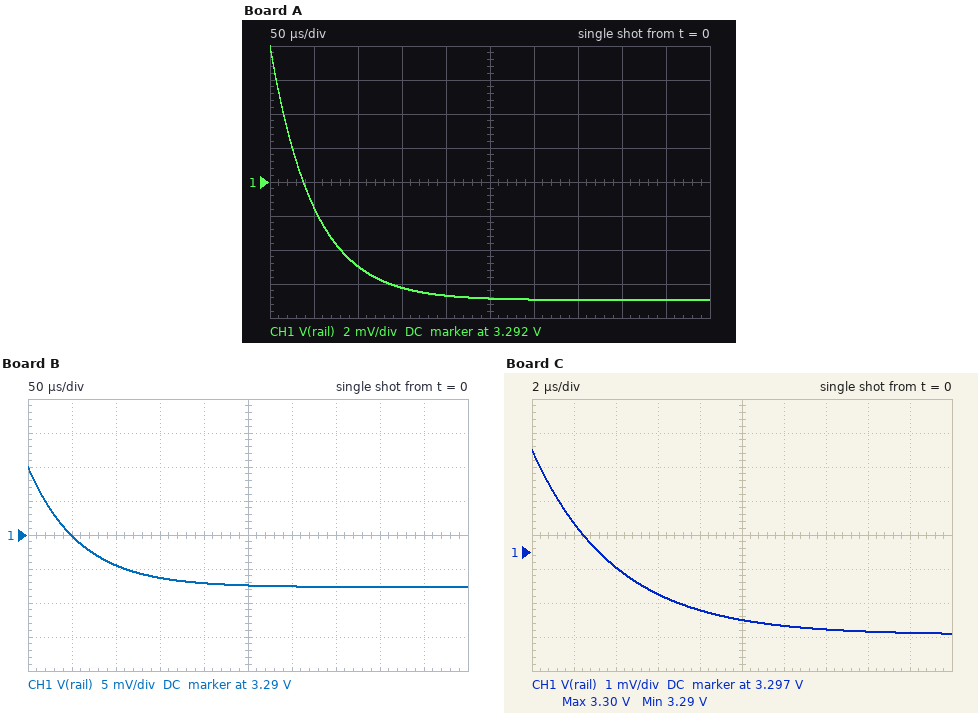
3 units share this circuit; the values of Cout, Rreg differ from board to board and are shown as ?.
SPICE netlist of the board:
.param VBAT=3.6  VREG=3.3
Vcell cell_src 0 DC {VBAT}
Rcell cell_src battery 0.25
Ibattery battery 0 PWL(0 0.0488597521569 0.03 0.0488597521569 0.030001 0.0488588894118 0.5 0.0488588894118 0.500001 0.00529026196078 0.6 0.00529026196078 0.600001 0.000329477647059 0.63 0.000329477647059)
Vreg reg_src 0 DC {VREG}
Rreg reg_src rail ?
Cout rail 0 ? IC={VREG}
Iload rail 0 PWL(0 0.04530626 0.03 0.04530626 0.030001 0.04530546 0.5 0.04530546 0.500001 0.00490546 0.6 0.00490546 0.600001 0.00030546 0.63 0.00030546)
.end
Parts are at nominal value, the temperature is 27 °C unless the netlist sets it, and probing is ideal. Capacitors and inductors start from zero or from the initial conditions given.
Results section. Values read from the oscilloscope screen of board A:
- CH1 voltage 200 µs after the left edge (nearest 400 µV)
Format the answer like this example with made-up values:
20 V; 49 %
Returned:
3.2852 V
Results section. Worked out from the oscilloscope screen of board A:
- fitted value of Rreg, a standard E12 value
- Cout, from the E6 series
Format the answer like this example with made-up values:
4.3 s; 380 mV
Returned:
0.33 Ω; 150 µF
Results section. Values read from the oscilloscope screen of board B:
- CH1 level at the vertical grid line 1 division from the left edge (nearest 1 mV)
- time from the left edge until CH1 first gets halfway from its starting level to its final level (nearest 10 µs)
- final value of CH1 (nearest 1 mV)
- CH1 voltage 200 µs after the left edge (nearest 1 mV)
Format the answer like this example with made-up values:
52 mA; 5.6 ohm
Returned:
3.290 V; 40 µs; 3.282 V; 3.283 V
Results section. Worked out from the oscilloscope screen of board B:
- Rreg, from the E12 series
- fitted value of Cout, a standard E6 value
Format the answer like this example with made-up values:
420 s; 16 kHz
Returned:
0.39 Ω; 150 µF
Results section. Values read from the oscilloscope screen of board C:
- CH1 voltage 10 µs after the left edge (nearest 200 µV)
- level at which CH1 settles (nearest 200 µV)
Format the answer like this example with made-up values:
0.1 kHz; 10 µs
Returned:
3.2950 V; 3.2946 V
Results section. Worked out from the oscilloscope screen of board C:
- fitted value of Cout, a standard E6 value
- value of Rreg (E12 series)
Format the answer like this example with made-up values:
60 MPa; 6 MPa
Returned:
33 µF; 0.12 Ω
